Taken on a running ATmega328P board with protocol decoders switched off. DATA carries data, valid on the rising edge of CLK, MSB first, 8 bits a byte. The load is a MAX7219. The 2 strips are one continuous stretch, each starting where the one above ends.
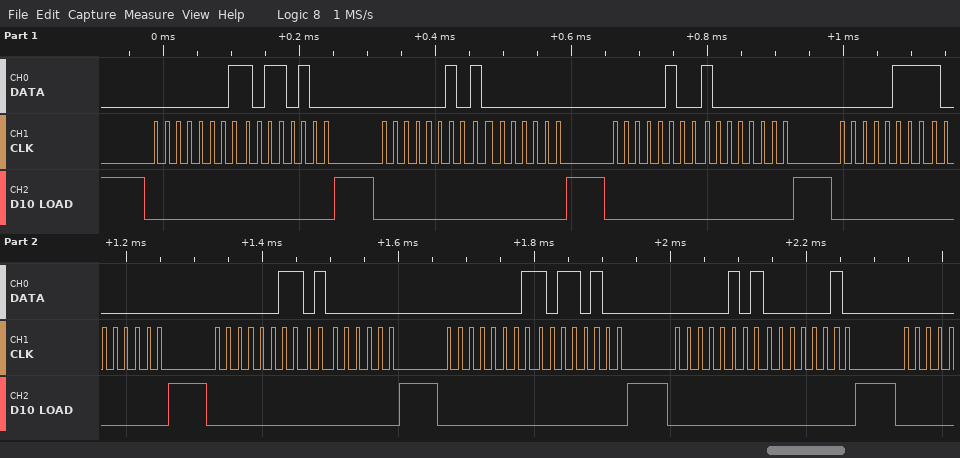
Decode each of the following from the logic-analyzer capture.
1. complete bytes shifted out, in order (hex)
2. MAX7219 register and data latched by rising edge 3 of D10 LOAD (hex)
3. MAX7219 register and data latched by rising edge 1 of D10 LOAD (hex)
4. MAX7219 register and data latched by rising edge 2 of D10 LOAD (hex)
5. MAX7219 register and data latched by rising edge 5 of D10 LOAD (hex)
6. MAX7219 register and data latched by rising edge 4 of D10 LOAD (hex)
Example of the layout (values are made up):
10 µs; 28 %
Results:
01 B4 02 80 04 80 07 80 03 40 01 B4 05 02; register 0x4, data 0x80; register 0x1, data 0xB4; register 0x2, data 0x80; register 0x3, data 0x40; register 0x7, data 0x80
